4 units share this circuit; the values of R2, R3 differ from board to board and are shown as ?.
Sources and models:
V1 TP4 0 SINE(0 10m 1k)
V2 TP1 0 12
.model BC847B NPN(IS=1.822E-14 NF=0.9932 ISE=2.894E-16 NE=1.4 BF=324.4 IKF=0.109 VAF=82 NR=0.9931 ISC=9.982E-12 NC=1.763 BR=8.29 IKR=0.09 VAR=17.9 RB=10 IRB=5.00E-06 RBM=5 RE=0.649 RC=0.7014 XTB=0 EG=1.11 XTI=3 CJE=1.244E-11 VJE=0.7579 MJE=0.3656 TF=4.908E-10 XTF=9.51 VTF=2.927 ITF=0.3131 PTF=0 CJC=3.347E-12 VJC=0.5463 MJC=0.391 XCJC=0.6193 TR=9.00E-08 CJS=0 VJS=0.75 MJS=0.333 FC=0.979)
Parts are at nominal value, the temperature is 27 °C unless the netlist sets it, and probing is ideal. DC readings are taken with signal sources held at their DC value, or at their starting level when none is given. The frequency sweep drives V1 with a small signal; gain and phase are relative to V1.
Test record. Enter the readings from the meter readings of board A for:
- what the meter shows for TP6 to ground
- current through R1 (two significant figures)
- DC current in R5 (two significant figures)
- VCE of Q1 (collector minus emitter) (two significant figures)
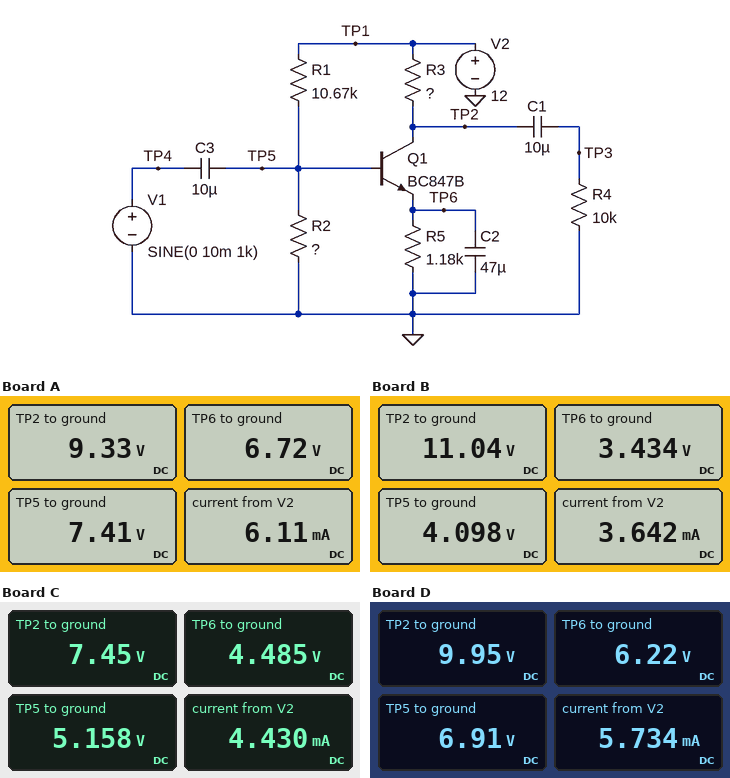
6.72 V
430 µA
5.7 mA
2.6 V
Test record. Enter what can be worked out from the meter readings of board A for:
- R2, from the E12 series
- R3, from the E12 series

18 kΩ
470 Ω
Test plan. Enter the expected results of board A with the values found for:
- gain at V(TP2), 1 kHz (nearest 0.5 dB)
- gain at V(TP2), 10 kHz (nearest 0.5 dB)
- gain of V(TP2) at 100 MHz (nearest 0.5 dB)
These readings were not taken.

36.5 dB
38.0 dB
34.0 dB
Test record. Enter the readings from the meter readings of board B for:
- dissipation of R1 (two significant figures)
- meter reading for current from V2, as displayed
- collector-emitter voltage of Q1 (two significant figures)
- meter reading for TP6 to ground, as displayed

5.9 mW
3.642 mA
7.6 V
3.434 V
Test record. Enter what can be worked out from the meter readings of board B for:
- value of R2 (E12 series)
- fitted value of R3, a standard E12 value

5.6 kΩ
330 Ω
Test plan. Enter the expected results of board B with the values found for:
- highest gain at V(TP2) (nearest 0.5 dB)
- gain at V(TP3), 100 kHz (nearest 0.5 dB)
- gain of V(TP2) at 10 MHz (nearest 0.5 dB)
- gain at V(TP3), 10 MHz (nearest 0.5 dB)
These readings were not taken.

30.0 dB
30.0 dB
30.0 dB
30.0 dB
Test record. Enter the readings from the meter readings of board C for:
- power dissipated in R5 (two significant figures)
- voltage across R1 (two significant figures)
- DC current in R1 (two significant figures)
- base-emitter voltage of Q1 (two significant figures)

17 mW
6.8 V
640 µA
670 mV
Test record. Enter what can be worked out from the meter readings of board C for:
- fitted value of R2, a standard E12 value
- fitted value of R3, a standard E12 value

8.2 kΩ
1.2 kΩ
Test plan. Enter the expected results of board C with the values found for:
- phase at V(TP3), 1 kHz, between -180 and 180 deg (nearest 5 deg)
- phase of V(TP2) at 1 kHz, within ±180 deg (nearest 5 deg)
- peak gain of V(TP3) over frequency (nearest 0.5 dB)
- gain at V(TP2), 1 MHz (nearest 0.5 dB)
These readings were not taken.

-155 deg
-155 deg
42.5 dB
42.5 dB
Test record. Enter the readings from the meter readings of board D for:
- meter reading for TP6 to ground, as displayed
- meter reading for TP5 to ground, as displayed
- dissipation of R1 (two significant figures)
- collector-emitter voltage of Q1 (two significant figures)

6.22 V
6.91 V
2.4 mW
3.7 V
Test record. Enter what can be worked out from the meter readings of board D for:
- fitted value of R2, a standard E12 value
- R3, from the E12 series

15 kΩ
390 Ω
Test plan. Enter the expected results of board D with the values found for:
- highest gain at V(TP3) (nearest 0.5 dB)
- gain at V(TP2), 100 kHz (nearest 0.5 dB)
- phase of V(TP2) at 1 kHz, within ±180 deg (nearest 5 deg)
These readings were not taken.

36.0 dB
36.0 dB
-150 deg
